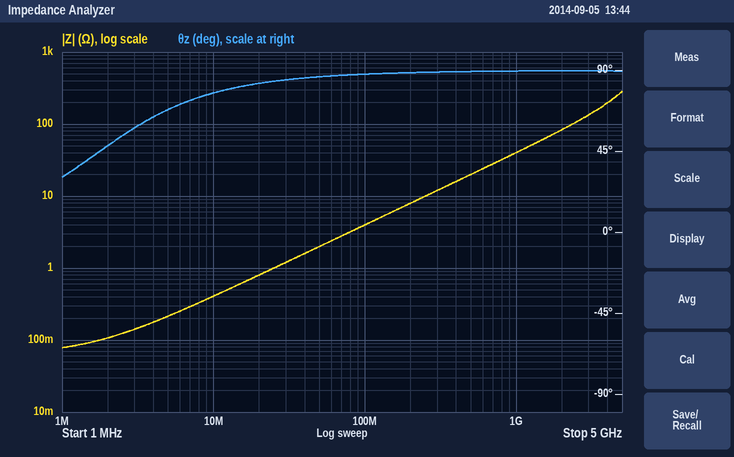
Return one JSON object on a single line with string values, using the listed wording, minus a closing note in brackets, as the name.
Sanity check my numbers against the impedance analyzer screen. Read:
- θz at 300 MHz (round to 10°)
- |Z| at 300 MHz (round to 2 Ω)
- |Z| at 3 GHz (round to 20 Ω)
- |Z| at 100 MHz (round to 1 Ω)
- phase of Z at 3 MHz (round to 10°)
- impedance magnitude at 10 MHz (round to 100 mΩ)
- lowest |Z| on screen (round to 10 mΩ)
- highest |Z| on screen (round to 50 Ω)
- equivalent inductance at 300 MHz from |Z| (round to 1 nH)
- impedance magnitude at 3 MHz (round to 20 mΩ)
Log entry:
{"θz at 300 MHz": "90°", "|Z| at 300 MHz": "12 Ω", "|Z| at 3 GHz": "140 Ω", "|Z| at 100 MHz": "4 Ω", "phase of Z at 3 MHz": "60°", "impedance magnitude at 10 MHz": "400 mΩ", "lowest |Z| on screen": "80 mΩ", "highest |Z| on screen": "300 Ω", "equivalent inductance at 300 MHz from |Z|": "6 nH", "impedance magnitude at 3 MHz": "140 mΩ"}
